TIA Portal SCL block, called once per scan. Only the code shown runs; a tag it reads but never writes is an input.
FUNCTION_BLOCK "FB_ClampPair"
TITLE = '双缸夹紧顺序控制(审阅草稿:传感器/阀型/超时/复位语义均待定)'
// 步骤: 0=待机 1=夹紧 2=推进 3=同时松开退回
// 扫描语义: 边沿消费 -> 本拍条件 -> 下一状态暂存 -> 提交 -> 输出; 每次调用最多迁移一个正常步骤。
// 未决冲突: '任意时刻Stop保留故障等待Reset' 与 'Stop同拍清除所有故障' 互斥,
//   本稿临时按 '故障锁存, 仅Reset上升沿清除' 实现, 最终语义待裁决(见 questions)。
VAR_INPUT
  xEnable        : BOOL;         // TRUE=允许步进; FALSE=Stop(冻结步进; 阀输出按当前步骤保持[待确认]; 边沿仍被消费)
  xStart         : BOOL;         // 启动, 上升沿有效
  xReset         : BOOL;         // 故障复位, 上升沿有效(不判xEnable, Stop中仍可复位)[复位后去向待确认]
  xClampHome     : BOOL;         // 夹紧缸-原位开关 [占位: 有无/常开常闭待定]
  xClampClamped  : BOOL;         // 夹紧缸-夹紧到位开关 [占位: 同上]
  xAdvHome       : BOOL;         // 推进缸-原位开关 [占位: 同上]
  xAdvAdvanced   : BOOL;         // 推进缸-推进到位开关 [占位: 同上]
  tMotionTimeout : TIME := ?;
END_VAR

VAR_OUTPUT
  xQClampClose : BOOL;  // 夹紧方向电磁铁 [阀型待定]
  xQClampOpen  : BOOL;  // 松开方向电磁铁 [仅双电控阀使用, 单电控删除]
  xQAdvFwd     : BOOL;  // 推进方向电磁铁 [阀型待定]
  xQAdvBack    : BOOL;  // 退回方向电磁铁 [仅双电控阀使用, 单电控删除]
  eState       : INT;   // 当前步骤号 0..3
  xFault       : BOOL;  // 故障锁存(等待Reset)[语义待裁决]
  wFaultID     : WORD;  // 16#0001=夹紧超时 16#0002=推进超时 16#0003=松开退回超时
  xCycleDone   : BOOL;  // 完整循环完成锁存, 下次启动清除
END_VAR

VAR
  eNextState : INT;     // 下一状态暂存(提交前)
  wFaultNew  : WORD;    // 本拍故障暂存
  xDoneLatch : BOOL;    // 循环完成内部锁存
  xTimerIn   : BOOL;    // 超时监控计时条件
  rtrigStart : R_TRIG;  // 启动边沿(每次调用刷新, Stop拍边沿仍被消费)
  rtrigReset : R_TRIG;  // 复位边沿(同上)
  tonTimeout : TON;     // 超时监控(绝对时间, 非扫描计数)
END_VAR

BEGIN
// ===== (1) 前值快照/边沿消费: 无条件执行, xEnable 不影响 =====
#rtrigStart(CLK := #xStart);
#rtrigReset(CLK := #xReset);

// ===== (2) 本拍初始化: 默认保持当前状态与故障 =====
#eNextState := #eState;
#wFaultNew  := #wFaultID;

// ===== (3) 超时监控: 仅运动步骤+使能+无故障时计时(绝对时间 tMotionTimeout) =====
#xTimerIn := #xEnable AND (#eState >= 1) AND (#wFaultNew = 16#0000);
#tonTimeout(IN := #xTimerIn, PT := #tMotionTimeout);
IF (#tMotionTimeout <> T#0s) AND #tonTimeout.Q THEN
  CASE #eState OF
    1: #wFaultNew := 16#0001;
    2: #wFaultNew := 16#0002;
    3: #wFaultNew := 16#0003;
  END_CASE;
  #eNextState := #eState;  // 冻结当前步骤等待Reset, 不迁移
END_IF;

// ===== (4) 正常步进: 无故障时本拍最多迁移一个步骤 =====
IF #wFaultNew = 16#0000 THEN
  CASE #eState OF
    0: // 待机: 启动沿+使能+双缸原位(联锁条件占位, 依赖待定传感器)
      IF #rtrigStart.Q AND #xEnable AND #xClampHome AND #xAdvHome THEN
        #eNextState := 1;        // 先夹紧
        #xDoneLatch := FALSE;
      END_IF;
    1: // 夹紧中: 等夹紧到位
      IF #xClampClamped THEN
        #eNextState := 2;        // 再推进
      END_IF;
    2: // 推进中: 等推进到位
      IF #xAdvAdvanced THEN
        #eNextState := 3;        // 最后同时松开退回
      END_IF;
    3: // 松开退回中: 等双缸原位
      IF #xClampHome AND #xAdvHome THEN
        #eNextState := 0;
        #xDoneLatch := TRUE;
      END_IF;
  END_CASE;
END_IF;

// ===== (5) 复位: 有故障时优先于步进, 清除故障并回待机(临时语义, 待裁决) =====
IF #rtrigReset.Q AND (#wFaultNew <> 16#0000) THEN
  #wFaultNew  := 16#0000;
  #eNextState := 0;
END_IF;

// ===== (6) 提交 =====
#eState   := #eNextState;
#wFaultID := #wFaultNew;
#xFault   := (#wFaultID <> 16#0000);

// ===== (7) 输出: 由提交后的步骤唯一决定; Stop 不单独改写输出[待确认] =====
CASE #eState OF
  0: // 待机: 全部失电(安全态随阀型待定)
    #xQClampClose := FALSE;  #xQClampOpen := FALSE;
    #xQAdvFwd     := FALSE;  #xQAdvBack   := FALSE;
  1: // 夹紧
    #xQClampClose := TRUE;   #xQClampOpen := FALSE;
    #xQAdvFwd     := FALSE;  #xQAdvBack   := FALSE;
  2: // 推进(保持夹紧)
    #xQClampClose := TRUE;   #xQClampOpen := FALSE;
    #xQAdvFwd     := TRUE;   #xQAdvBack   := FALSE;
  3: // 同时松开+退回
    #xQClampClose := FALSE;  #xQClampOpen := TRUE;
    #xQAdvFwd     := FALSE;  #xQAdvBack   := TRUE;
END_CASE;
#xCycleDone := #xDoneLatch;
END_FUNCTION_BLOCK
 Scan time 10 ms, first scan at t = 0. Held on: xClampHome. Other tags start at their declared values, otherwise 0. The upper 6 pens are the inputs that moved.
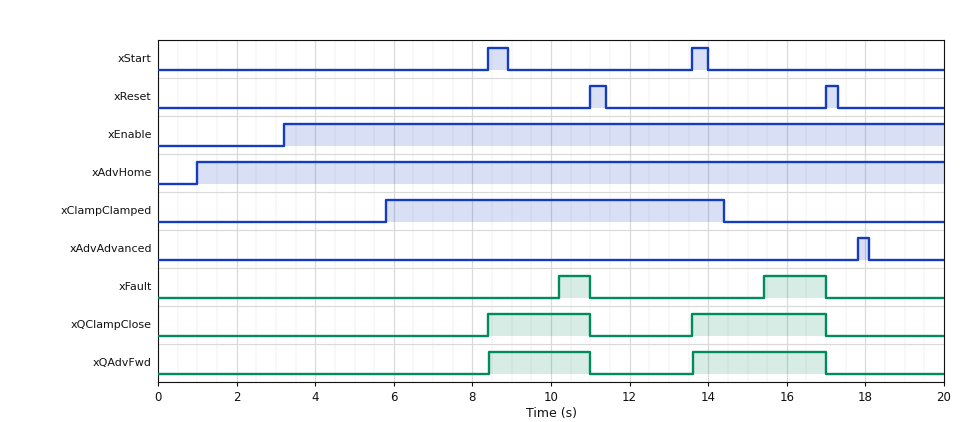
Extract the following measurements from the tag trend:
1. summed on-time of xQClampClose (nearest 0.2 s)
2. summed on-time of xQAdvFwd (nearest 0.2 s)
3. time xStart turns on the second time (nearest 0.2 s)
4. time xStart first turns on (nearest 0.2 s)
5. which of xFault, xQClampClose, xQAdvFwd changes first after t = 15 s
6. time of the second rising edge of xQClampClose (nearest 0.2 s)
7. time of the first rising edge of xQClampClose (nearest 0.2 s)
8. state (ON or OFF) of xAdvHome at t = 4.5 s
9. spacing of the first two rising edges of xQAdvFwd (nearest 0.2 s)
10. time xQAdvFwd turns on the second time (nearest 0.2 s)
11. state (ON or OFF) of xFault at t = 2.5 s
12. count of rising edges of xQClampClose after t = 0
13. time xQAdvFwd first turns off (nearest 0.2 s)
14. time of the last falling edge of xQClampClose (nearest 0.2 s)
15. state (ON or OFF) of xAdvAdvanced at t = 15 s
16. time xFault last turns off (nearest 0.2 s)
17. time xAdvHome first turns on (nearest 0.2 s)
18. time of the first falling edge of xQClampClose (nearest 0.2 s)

6.0 s
6.0 s
13.6 s
8.4 s
xFault
13.6 s
8.4 s
ON
5.2 s
13.6 s
OFF
2
11.0 s
17.0 s
OFF
17.0 s
1.0 s
11.0 s
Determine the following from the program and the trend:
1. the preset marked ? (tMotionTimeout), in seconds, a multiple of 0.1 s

1.8 s
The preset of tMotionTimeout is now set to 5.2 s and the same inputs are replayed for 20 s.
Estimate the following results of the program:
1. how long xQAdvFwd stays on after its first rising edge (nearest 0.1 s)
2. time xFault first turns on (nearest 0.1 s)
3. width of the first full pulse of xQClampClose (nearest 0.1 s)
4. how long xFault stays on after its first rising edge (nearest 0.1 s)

8.6 s
13.6 s
8.6 s
3.4 s
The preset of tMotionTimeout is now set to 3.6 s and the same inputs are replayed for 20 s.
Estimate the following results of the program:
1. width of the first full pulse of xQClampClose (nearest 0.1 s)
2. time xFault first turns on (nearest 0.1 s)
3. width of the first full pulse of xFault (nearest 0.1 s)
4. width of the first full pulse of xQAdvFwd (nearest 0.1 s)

8.6 s
12.0 s
5.0 s
8.6 s
